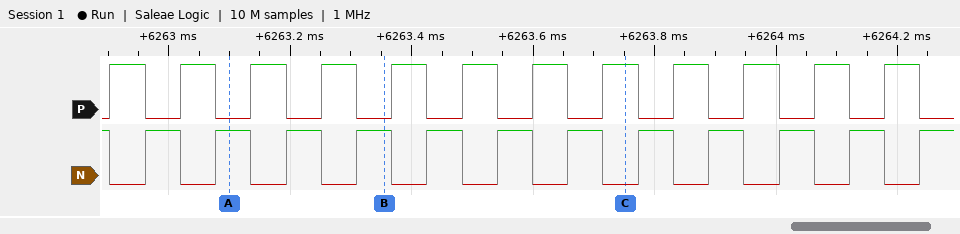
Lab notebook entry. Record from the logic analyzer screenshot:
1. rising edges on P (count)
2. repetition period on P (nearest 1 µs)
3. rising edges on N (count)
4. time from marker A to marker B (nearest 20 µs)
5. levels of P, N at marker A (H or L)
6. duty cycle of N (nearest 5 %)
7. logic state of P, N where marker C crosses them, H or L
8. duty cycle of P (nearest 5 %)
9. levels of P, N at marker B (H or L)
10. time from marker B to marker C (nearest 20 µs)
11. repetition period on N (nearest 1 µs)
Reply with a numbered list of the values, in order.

1. 12
2. 116 µs
3. 12
4. 260 µs
5. P=L, N=H
6. 50 %
7. P=H, N=L
8. 50 %
9. P=L, N=H
10. 400 µs
11. 116 µs
